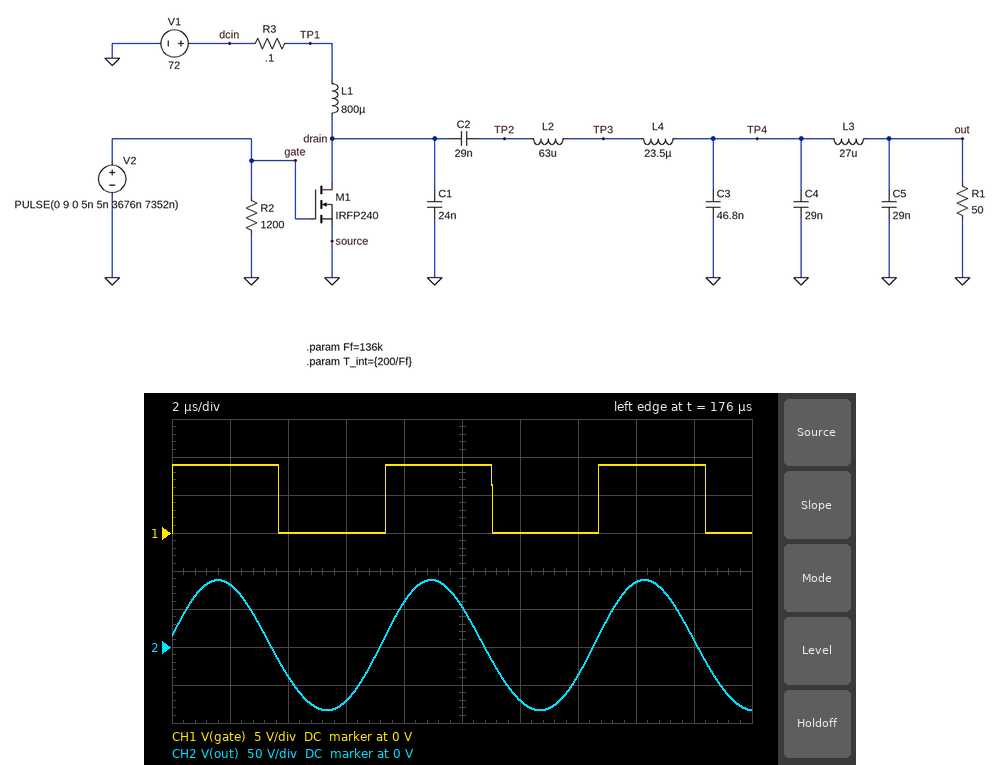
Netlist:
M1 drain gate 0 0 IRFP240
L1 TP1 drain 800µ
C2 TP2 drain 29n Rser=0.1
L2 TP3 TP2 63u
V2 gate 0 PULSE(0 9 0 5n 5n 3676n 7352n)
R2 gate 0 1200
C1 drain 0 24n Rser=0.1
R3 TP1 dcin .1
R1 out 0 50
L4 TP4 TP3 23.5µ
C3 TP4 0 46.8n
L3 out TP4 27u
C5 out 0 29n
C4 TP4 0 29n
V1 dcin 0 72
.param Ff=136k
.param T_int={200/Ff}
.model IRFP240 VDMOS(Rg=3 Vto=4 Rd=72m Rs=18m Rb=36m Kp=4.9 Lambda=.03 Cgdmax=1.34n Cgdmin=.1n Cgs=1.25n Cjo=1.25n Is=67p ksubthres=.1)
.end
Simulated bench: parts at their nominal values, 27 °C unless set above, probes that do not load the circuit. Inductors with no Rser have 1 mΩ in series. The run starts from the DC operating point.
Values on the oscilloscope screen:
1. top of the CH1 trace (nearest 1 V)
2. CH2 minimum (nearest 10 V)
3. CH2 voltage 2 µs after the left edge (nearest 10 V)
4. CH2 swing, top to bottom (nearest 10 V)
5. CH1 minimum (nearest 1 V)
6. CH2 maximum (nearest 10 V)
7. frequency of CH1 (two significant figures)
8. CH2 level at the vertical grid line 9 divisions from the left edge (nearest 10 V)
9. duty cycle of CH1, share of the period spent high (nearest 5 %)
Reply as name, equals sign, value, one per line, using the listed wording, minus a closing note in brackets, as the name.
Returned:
top of the CH1 trace = 9 V
CH2 minimum = -80 V
CH2 voltage 2 µs after the left edge = 80 V
CH2 swing, top to bottom = 170 V
CH1 minimum = 0 V
CH2 maximum = 90 V
frequency of CH1 = 140 kHz
CH2 level at the vertical grid line 9 divisions from the left edge = 10 V
duty cycle of CH1, share of the period spent high = 50 %
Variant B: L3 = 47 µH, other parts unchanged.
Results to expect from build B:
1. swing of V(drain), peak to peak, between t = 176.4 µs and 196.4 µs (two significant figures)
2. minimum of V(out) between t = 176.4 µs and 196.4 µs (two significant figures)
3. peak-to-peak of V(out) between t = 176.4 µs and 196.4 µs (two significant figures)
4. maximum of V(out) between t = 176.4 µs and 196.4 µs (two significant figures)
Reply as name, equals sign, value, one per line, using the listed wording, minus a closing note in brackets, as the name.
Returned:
swing of V(drain), peak to peak, between t = 176.4 µs and 196.4 µs = 230 V
minimum of V(out) between t = 176.4 µs and 196.4 µs = -130 V
peak-to-peak of V(out) between t = 176.4 µs and 196.4 µs = 250 V
maximum of V(out) between t = 176.4 µs and 196.4 µs = 130 V
